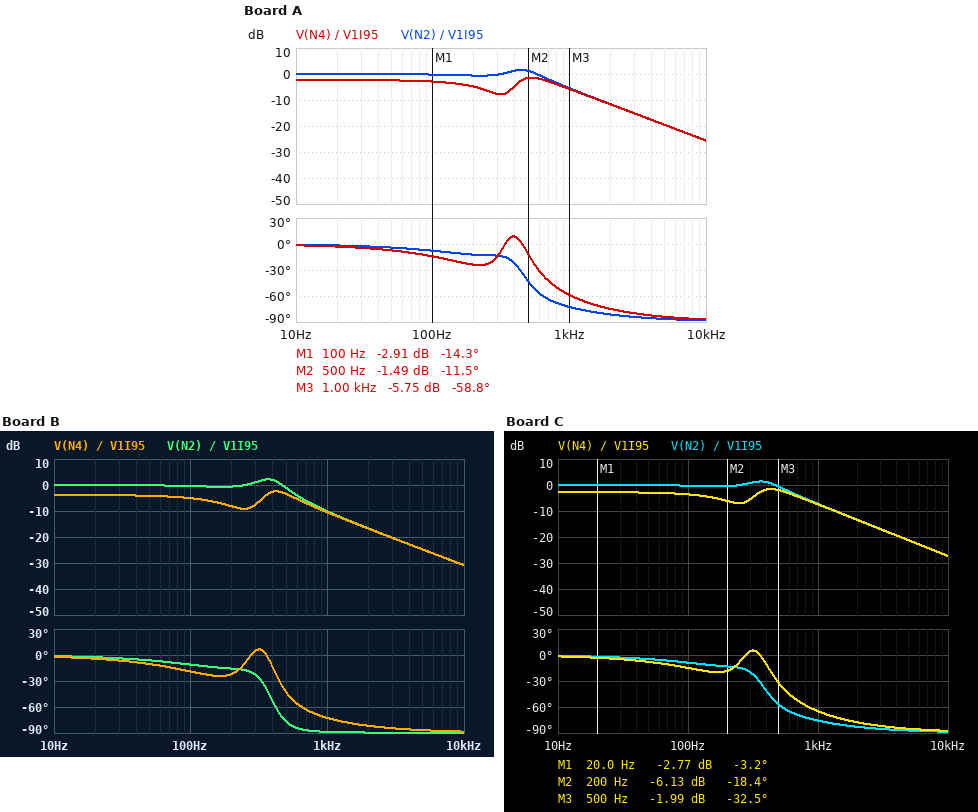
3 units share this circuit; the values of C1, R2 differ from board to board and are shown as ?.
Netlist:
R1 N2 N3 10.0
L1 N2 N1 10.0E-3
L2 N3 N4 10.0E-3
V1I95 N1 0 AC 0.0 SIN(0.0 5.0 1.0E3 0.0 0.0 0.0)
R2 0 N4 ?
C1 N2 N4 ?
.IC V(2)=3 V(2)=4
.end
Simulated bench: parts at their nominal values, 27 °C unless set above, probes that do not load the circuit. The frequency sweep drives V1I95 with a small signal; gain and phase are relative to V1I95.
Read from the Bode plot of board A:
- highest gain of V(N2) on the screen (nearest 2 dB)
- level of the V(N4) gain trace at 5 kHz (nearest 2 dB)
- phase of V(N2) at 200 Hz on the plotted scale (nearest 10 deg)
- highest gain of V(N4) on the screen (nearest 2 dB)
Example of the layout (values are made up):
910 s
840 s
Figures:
2 dB
-20 dB
-10 deg
-2 dB
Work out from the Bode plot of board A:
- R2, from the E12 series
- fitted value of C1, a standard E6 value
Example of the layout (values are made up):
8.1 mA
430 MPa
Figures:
33 Ω
22 µF
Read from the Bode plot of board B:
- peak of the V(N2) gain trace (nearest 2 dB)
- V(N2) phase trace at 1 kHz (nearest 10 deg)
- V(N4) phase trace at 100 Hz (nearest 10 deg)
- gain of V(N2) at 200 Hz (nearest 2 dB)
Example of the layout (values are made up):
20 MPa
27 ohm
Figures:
2 dB
-90 deg
-20 deg
0 dB
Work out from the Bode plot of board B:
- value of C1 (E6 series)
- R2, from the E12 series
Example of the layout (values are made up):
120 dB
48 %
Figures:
33 µF
18 Ω
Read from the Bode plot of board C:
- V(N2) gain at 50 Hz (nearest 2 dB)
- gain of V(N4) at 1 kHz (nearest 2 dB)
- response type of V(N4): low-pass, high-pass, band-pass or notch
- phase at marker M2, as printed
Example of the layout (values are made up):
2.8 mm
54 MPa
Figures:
0 dB
-8 dB
low-pass
-18.4 deg
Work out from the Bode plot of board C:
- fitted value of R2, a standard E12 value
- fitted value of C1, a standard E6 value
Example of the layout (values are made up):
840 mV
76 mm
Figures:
27 Ω
33 µF
